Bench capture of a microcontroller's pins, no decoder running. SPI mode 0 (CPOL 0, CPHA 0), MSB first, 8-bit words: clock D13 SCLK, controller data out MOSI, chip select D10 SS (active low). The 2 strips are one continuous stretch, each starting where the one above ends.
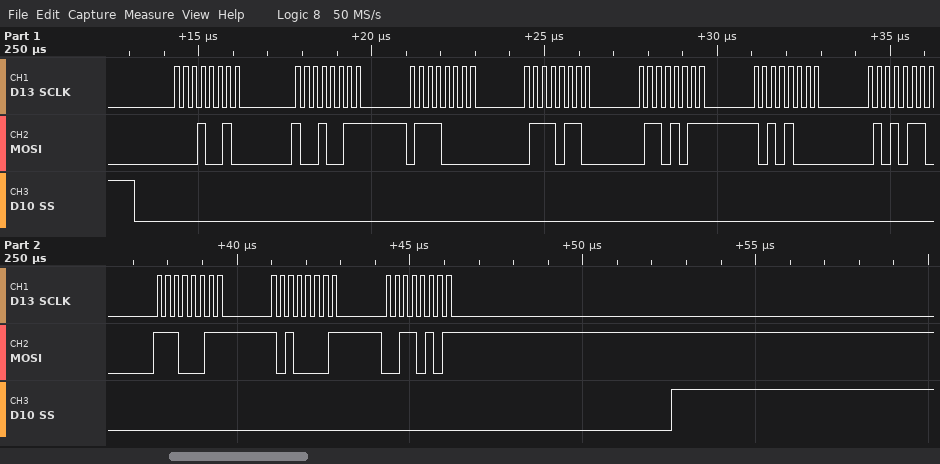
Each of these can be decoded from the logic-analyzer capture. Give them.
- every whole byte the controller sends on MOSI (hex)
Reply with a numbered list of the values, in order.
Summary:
1. 12 93 70 76 6B A8 56 E3 A1 35
